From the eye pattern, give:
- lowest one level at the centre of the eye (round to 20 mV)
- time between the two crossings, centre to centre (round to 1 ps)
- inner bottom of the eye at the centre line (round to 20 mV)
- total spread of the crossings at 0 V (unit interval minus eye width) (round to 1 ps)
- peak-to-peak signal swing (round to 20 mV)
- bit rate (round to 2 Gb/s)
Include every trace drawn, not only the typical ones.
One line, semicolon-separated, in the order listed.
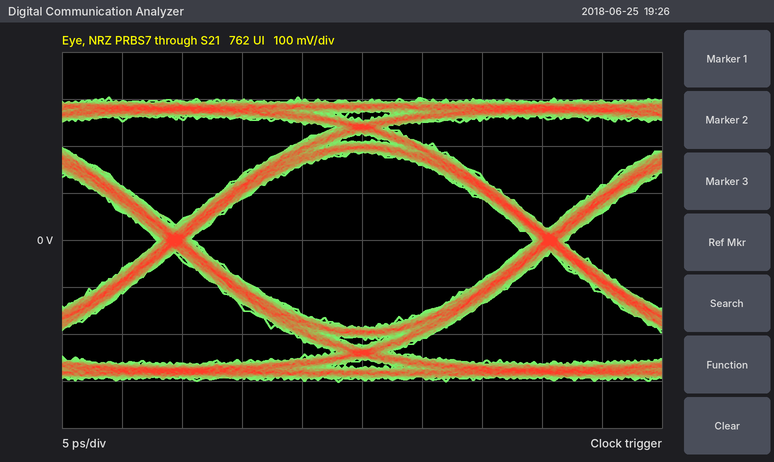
180 mV; 31 ps; -180 mV; 3 ps; 600 mV; 32 Gb/s
